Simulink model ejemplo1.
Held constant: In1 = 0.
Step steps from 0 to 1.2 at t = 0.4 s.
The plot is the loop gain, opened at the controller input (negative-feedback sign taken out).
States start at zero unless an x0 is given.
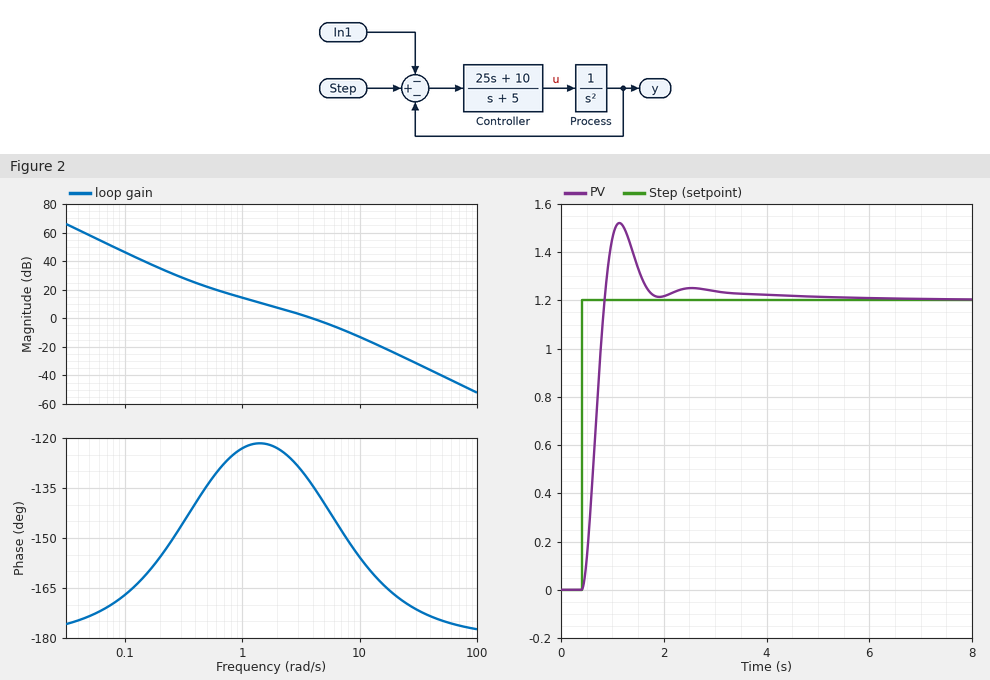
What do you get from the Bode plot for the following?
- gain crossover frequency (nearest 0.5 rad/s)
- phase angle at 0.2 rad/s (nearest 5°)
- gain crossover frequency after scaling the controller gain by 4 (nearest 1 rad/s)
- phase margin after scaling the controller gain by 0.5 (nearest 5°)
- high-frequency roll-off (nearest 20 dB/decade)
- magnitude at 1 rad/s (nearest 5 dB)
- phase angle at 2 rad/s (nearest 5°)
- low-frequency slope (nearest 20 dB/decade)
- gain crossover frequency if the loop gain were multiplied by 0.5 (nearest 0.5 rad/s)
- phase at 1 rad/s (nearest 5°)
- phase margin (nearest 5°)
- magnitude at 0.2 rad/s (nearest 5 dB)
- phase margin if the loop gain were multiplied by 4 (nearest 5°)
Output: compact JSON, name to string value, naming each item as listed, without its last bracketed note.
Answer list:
{"gain crossover frequency": "4.0 rad/s", "phase angle at 0.2 rad/s": "-155°", "gain crossover frequency after scaling the controller gain by 4": "9 rad/s", "phase margin after scaling the controller gain by 0.5": "55°", "high-frequency roll-off": "-40 dB/decade", "magnitude at 1 rad/s": "15 dB", "phase angle at 2 rad/s": "-125°", "low-frequency slope": "-40 dB/decade", "gain crossover frequency if the loop gain were multiplied by 0.5": "2.5 rad/s", "phase at 1 rad/s": "-125°", "phase margin": "45°", "magnitude at 0.2 rad/s": "35 dB", "phase margin if the loop gain were multiplied by 4": "25°"}
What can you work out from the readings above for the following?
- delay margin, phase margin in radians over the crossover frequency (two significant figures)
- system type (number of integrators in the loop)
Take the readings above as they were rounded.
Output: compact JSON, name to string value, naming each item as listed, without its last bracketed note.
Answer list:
{"delay margin, phase margin in radians over the crossover frequency": "0.20 s", "system type": "2"}
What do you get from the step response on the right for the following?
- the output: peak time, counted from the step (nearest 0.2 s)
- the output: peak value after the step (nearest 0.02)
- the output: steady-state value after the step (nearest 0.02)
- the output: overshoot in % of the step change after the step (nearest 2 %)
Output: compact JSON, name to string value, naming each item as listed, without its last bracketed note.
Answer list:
{"the output: peak time, counted from the step": "0.8 s", "the output: peak value after the step": "1.52", "the output: steady-state value after the step": "1.20", "the output: overshoot in % of the step change after the step": "26 %"}
